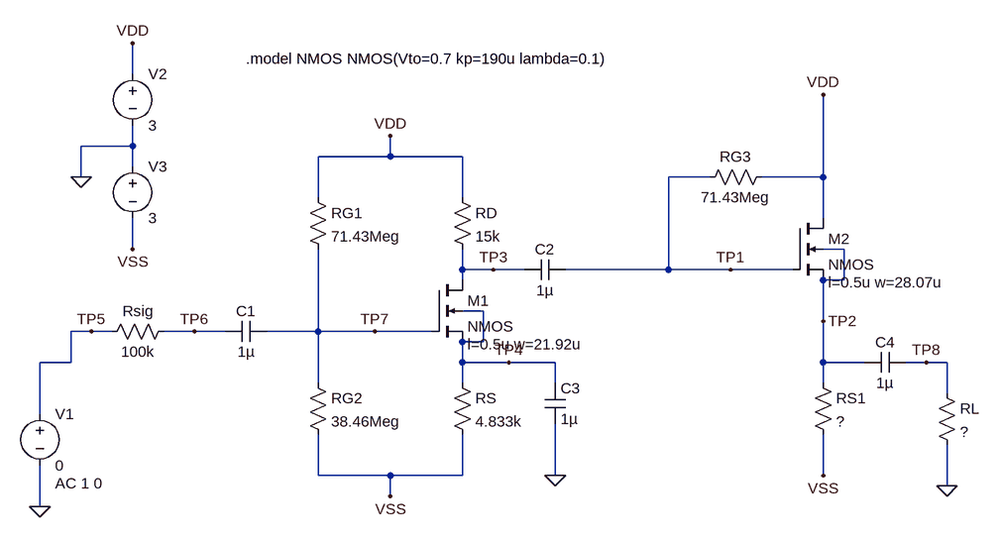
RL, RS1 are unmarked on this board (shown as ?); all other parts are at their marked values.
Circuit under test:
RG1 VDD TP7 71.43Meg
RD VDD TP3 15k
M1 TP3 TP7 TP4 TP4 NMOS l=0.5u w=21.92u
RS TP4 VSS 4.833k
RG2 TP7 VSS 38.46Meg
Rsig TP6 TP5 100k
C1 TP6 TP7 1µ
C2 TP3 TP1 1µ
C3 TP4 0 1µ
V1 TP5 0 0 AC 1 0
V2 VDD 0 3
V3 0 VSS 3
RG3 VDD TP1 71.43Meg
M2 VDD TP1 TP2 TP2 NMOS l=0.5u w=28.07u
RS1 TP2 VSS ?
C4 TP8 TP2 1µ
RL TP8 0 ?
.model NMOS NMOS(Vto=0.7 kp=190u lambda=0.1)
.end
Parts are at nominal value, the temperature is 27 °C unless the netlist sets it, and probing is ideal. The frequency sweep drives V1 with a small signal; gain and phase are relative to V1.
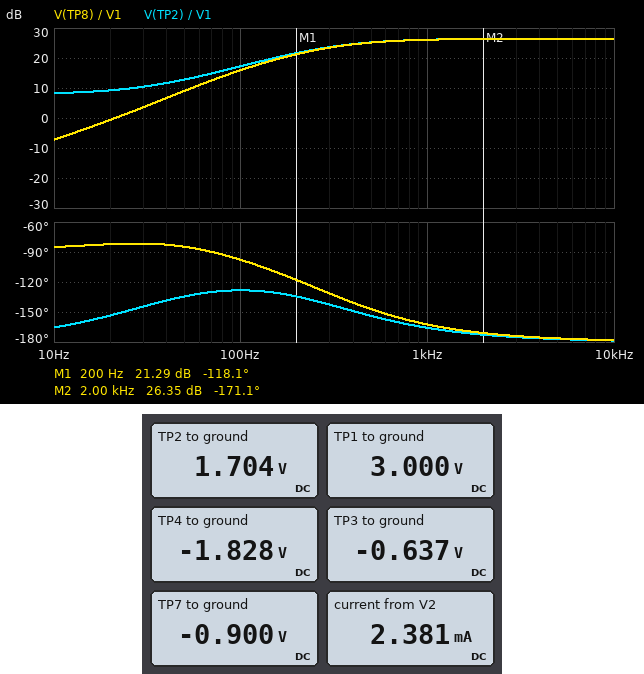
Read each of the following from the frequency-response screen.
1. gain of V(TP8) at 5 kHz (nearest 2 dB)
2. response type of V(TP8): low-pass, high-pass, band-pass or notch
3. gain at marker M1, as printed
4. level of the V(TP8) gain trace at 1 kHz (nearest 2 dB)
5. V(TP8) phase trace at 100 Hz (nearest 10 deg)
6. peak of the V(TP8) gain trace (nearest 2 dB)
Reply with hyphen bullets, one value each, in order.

- 26 dB
- high-pass
- 21.29 dB
- 26 dB
- -100 deg
- 26 dB
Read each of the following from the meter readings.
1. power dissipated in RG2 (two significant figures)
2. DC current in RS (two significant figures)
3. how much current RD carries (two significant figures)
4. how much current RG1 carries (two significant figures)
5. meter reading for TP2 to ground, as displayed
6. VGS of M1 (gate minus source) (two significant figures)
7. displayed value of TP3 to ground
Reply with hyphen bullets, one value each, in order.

- 110 nW
- 240 µA
- 240 µA
- 55 nA
- 1.704 V
- 930 mV
- -0.637 V
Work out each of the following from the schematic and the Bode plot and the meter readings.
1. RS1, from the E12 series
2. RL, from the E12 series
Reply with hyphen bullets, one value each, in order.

- 2.2 kΩ
- 2.7 kΩ
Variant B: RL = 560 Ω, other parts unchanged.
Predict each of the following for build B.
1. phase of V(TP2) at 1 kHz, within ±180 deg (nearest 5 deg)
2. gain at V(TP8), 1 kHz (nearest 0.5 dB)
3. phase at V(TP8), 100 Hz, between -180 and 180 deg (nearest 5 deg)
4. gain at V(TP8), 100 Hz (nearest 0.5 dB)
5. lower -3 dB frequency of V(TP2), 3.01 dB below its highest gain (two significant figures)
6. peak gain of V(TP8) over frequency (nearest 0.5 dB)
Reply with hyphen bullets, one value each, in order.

- -170 deg
- 24.5 dB
- -60 deg
- 7.5 dB
- 230 Hz
- 25.0 dB
